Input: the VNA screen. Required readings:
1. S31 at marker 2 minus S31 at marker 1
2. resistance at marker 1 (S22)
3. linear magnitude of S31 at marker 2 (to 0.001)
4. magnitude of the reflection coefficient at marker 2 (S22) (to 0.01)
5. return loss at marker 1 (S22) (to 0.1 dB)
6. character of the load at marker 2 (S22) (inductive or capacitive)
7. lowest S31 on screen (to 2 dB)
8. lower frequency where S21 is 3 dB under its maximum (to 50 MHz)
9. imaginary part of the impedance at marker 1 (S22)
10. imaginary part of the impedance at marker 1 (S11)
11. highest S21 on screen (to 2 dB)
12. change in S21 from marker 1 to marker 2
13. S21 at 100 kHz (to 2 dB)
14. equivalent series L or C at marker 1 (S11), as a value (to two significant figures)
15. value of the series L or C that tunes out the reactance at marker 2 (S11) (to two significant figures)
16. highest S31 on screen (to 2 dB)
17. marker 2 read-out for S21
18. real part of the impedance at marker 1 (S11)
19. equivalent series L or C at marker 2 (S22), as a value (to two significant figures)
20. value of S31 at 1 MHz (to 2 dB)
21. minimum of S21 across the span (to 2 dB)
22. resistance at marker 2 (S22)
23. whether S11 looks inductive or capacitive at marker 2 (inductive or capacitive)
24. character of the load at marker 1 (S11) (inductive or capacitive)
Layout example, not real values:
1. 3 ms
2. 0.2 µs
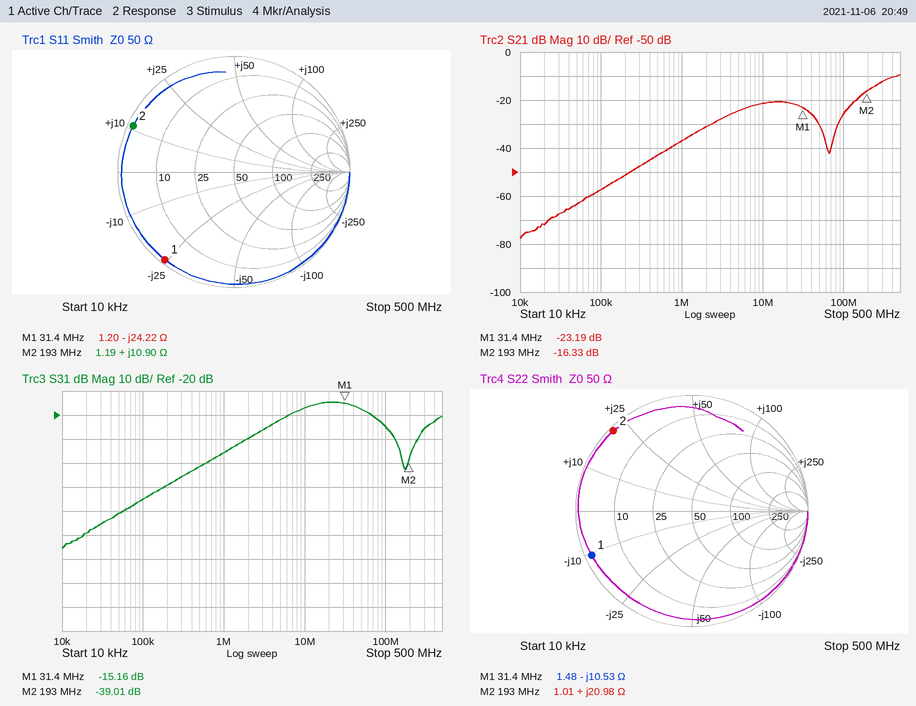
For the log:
1. -23.85 dB
2. 1.48 Ω
3. 0.011
4. 0.97
5. 0.5 dB
6. inductive
7. -76 dB
8. 300 MHz
9. -10.53 Ω
10. -24.22 Ω
11. -10 dB
12. 6.86 dB
13. -58 dB
14. 210 pF
15. 76 pF
16. -14 dB
17. -16.33 dB
18. 1.20 Ω
19. 17 nH
20. -36 dB
21. -78 dB
22. 1.01 Ω
23. inductive
24. capacitive
